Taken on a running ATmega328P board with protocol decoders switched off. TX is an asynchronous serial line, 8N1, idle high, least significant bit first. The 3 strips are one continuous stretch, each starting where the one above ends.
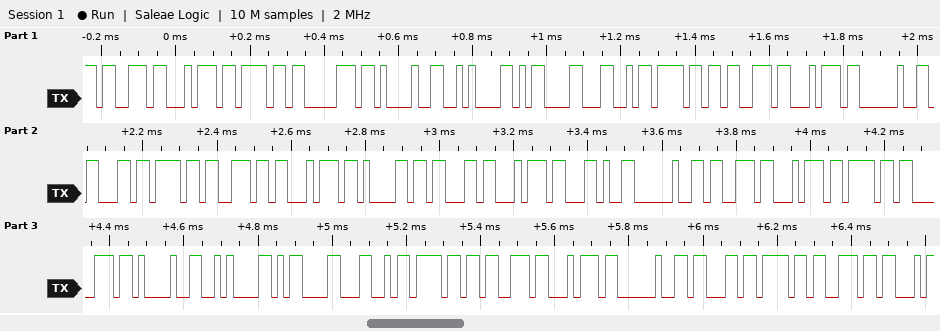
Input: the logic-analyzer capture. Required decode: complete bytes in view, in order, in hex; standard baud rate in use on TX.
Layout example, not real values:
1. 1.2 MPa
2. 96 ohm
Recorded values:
1. 73 74 6F 70 21 0A 0D 4C 6F 73 74 20 63 6F 6E 74 61 63 74 2C 20 73 74 6F 70 21 0A 0D 4C 6F 73 74 20 63 6F 6E
2. 57600 baud
